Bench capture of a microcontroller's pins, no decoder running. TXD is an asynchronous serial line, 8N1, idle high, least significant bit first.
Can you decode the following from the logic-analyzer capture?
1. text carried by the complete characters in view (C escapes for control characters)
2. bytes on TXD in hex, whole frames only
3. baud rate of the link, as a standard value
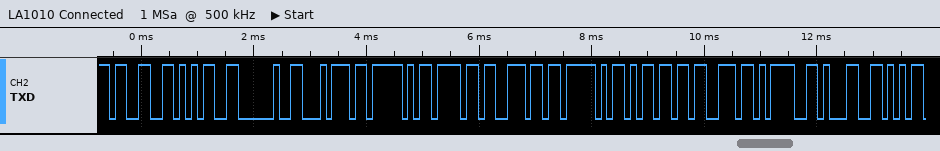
"35 t_on_ms=1"
33 35 20 74 5F 6F 6E 5F 6D 73 3D 31
9600 baud
